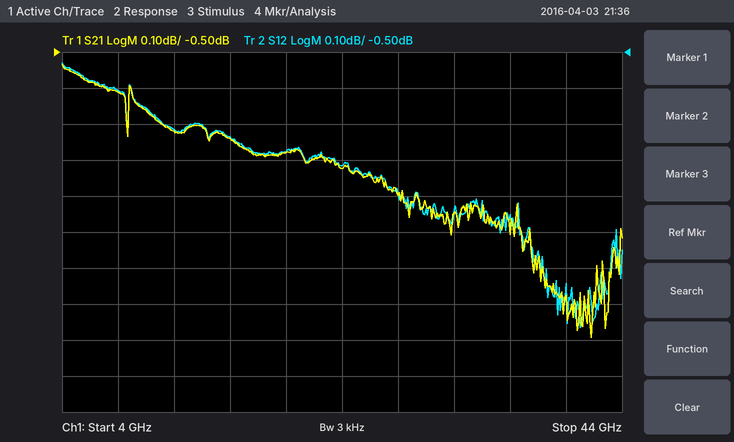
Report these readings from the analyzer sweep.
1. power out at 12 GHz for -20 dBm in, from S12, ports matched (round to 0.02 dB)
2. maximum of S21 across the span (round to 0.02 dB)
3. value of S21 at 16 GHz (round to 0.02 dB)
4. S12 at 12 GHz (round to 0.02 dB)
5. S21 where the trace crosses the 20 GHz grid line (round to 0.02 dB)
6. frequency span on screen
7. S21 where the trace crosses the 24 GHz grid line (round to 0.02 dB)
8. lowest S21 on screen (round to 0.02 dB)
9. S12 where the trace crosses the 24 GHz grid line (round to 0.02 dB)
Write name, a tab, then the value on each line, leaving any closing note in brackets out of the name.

power out at 12 GHz for -20 dBm in, from S12, ports matched	-20.72 dBm
maximum of S21 across the span	-0.54 dB
value of S21 at 16 GHz	-0.74 dB
S12 at 12 GHz	-0.72 dB
S21 where the trace crosses the 20 GHz grid line	-0.78 dB
frequency span on screen	40 GHz
S21 where the trace crosses the 24 GHz grid line	-0.82 dB
lowest S21 on screen	-1.30 dB
S12 where the trace crosses the 24 GHz grid line	-0.82 dB
